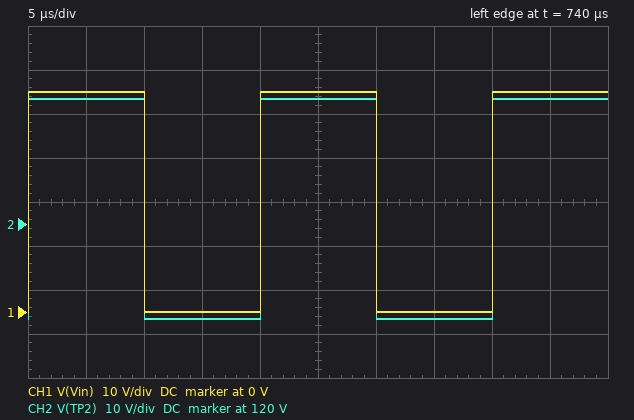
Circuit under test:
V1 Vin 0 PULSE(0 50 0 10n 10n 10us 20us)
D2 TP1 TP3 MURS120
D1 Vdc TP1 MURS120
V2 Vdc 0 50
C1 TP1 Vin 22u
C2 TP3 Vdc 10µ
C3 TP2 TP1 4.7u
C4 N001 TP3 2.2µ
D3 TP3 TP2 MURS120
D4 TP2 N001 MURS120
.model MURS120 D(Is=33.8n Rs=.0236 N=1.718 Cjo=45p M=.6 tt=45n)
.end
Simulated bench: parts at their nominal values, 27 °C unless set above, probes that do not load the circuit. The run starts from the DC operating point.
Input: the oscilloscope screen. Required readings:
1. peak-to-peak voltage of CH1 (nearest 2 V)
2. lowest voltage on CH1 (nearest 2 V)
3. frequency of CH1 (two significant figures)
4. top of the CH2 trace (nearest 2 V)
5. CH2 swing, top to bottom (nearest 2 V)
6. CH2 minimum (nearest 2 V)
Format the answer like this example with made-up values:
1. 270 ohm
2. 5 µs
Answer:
1. 50 V
2. 0 V
3. 50 kHz
4. 148 V
5. 50 V
6. 98 V
